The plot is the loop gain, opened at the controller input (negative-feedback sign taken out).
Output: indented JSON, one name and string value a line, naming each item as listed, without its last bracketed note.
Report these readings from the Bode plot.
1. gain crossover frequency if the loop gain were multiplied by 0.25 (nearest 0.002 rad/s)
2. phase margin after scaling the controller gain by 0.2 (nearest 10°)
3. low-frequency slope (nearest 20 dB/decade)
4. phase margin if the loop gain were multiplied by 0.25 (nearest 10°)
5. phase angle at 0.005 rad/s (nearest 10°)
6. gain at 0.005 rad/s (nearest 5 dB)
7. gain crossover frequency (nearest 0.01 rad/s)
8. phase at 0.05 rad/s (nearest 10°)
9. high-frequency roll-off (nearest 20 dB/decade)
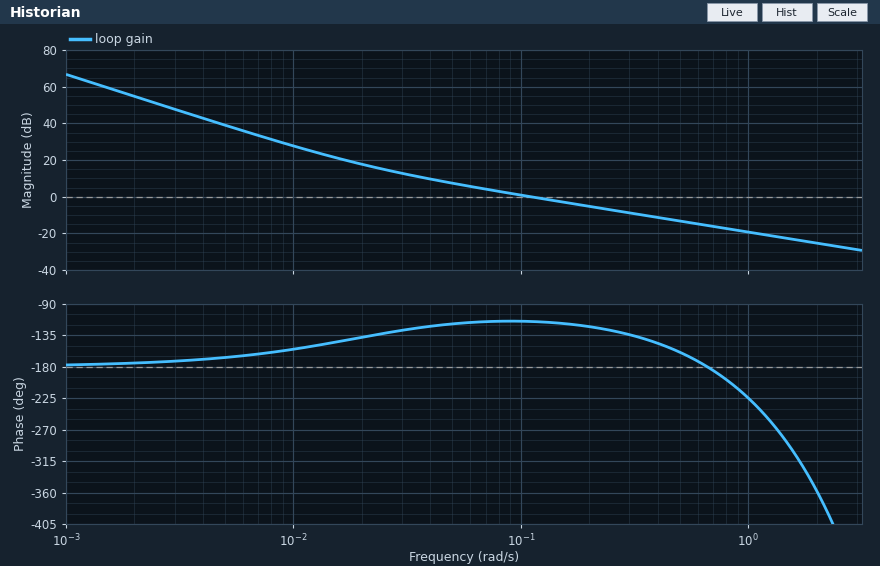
{
  "gain crossover frequency if the loop gain were multiplied by 0.25": "0.032 rad/s",
  "phase margin after scaling the controller gain by 0.2": "50°",
  "low-frequency slope": "-40 dB/decade",
  "phase margin if the loop gain were multiplied by 0.25": "50°",
  "phase angle at 0.005 rad/s": "-170°",
  "gain at 0.005 rad/s": "40 dB",
  "gain crossover frequency": "0.11 rad/s",
  "phase at 0.05 rad/s": "-120°",
  "high-frequency roll-off": "-20 dB/decade"
}
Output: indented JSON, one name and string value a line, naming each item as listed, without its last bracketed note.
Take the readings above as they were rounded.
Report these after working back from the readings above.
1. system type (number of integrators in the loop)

{
  "system type": "2"
}
